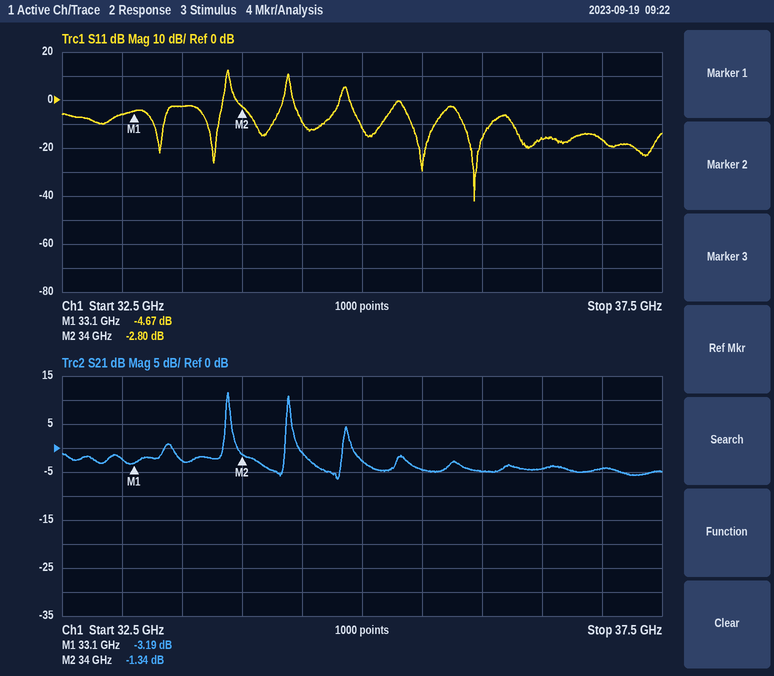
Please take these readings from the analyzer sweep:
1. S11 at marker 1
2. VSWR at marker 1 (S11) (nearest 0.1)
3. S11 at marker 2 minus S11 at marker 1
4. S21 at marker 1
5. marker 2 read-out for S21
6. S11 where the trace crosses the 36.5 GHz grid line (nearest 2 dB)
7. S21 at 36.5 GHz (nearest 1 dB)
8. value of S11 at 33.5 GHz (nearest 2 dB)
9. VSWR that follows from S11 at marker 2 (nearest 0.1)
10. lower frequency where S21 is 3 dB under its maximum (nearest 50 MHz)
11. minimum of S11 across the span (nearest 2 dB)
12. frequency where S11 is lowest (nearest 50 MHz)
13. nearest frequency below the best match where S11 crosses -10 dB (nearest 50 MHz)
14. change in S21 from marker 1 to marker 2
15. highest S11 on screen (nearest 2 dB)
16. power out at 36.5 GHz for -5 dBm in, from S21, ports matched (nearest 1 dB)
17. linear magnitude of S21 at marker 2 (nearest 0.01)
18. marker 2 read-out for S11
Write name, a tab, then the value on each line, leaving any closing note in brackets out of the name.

S11 at marker 1	-4.67 dB
VSWR at marker 1 (S11)	3.8
S11 at marker 2 minus S11 at marker 1	1.87 dB
S21 at marker 1	-3.19 dB
marker 2 read-out for S21	-1.34 dB
S11 where the trace crosses the 36.5 GHz grid line	-16 dB
S21 at 36.5 GHz	-4 dB
value of S11 at 33.5 GHz	-2 dB
VSWR that follows from S11 at marker 2	6.3
lower frequency where S21 is 3 dB under its maximum	33.85 GHz
minimum of S11 across the span	-42 dB
frequency where S11 is lowest	35.95 GHz
nearest frequency below the best match where S11 crosses -10 dB	35.85 GHz
change in S21 from marker 1 to marker 2	1.85 dB
highest S11 on screen	12 dB
power out at 36.5 GHz for -5 dBm in, from S21, ports matched	-9 dBm
linear magnitude of S21 at marker 2	0.86
marker 2 read-out for S11	-2.80 dB
